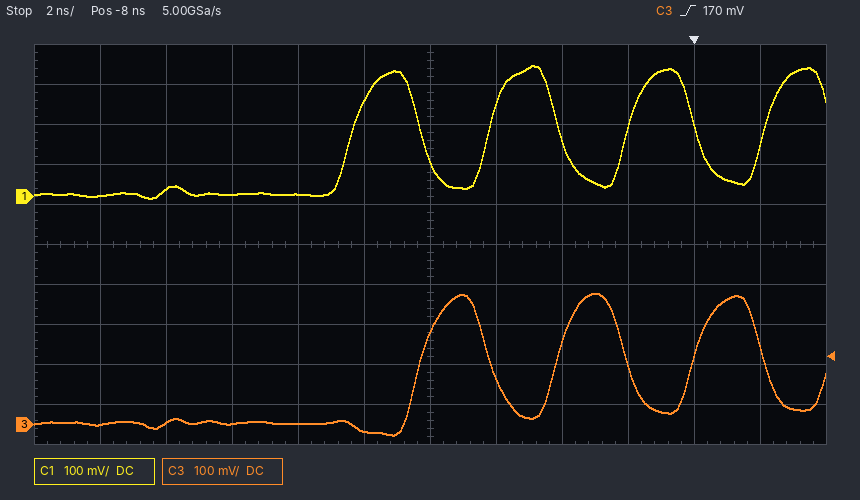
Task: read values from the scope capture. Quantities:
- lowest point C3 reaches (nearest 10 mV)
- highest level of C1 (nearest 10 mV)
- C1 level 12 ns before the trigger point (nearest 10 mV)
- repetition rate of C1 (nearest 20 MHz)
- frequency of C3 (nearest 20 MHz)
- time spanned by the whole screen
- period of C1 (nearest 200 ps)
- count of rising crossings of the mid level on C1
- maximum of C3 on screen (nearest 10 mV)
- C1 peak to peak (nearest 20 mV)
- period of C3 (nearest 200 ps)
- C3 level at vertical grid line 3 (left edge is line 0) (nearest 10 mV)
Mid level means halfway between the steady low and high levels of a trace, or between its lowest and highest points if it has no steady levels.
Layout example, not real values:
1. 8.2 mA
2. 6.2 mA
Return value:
1. -30 mV
2. 330 mV
3. 10 mV
4. 240 MHz
5. 240 MHz
6. 24 ns
7. 4.2 ns
8. 4
9. 330 mV
10. 340 mV
11. 4.2 ns
12. 0 mV
